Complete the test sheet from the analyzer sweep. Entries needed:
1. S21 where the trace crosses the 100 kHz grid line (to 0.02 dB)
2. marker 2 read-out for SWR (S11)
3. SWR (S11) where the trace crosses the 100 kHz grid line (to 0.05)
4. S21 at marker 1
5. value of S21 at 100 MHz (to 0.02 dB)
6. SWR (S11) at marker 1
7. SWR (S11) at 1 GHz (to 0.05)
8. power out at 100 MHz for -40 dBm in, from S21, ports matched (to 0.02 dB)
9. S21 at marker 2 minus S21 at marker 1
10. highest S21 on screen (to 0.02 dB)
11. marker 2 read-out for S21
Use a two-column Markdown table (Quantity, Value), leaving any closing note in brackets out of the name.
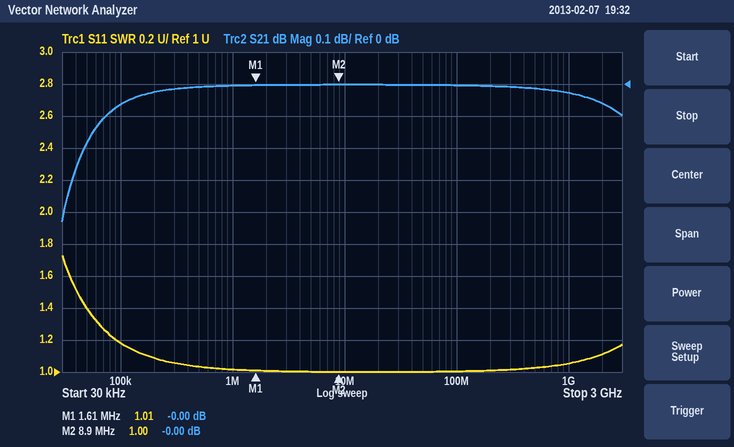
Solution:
| Quantity | Value |
|---|---|
| S21 where the trace crosses the 100 kHz grid line | -0.06 dB |
| marker 2 read-out for SWR | 1.00 |
| SWR (S11) where the trace crosses the 100 kHz grid line | 1.20 |
| S21 at marker 1 | -0.00 dB |
| value of S21 at 100 MHz | 0.00 dB |
| SWR (S11) at marker 1 | 1.01 |
| SWR (S11) at 1 GHz | 1.05 |
| power out at 100 MHz for -40 dBm in, from S21, ports matched | -40.00 dBm |
| S21 at marker 2 minus S21 at marker 1 | 0.00 dB |
| highest S21 on screen | 0.00 dB |
| marker 2 read-out for S21 | -0.00 dB |
